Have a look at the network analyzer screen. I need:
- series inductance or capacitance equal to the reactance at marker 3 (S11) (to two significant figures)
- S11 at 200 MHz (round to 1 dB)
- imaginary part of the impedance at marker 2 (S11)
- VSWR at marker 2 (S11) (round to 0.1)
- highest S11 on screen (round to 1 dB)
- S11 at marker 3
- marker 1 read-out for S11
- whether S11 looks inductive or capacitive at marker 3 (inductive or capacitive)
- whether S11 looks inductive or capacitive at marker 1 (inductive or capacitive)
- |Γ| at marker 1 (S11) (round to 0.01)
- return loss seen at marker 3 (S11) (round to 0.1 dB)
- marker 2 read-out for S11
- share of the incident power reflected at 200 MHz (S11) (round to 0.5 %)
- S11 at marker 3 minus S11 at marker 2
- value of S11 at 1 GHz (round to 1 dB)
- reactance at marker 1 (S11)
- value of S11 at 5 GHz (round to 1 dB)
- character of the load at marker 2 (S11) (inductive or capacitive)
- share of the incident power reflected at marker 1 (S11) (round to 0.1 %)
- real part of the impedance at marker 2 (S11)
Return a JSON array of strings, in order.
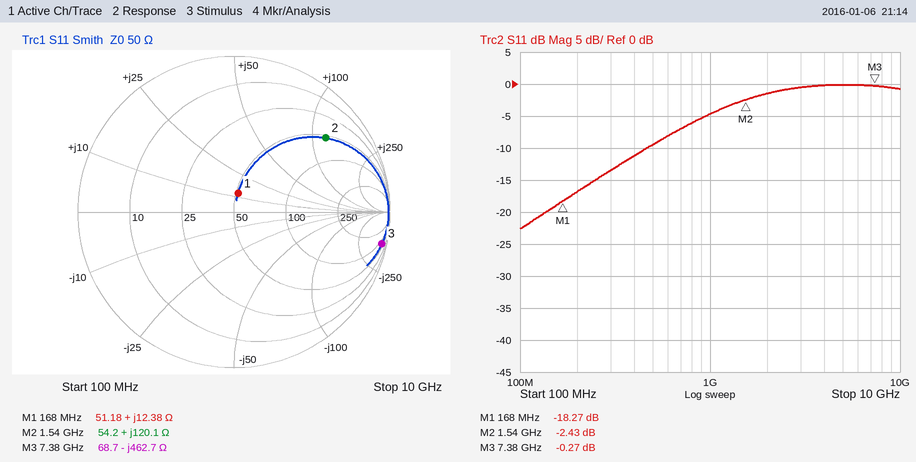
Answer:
["47 fF", "-17 dB", "+120.1 Ω", "7.2", "0 dB", "-0.27 dB", "-18.27 dB", "capacitive", "inductive", "0.12", "0.3 dB", "-2.43 dB", "2.0 %", "2.16 dB", "-5 dB", "+12.38 Ω", "0 dB", "inductive", "1.5 %", "54.2 Ω"]
